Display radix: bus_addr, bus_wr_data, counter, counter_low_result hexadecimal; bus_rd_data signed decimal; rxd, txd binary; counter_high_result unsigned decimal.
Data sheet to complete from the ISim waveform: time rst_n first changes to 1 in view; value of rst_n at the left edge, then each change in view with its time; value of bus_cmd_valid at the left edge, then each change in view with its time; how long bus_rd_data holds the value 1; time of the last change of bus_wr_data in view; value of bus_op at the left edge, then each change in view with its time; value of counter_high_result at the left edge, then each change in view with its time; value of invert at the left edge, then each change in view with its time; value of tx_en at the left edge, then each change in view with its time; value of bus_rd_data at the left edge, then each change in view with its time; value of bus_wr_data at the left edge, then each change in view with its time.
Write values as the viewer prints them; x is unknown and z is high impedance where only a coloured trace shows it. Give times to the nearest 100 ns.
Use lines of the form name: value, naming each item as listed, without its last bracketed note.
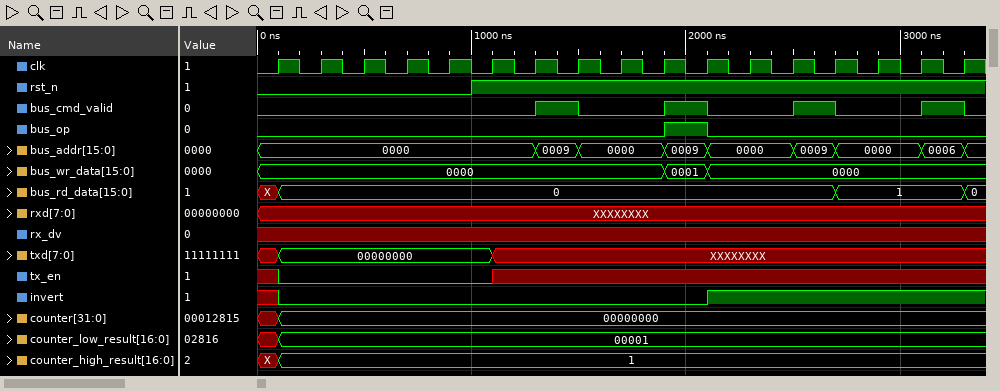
time rst_n first changes to 1 in view: 1000 ns
value of rst_n at the left edge, then each change in view with its time: 0, 1 at 1000 ns
value of bus_cmd_valid at the left edge, then each change in view with its time: 0, 1 at 1300 ns, 0 at 1500 ns, 1 at 1900 ns, 0 at 2100 ns, 1 at 2500 ns, 0 at 2700 ns, 1 at 3100 ns, 0 at 3300 ns
how long bus_rd_data holds the value 1: 600 ns
time of the last change of bus_wr_data in view: 2100 ns
value of bus_op at the left edge, then each change in view with its time: 0, 1 at 1900 ns, 0 at 2100 ns
value of counter_high_result at the left edge, then each change in view with its time: X, 1 at 100 ns
value of invert at the left edge, then each change in view with its time: x, 0 at 100 ns, 1 at 2100 ns
value of tx_en at the left edge, then each change in view with its time: x, 0 at 100 ns, x at 1100 ns
value of bus_rd_data at the left edge, then each change in view with its time: X, 0 at 100 ns, 1 at 2700 ns, 0 at 3300 ns
value of bus_wr_data at the left edge, then each change in view with its time: 0000, 0001 at 1900 ns, 0000 at 2100 ns
